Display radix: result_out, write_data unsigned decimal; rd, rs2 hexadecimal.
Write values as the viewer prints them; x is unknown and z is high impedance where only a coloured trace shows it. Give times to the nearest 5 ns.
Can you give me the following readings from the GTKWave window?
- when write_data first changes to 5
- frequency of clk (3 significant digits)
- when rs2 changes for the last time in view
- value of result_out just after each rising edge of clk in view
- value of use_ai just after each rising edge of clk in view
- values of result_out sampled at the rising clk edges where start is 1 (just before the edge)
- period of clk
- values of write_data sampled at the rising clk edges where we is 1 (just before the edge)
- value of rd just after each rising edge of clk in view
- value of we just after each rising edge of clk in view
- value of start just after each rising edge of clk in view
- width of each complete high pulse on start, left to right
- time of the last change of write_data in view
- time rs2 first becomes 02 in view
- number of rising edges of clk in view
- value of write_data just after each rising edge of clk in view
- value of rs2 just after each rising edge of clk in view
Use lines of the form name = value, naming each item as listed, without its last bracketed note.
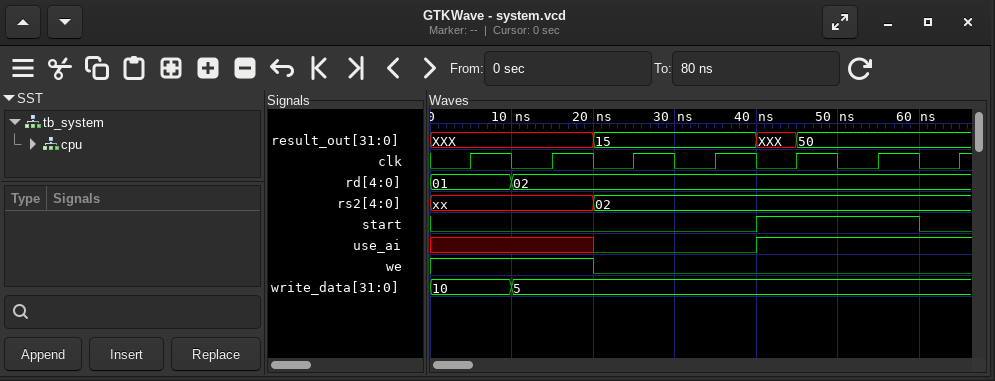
when write_data first changes to 5 = 10 ns
frequency of clk = 100 MHz
when rs2 changes for the last time in view = 20 ns
value of result_out just after each rising edge of clk in view = XXX, XXX, 15, 15, 50, 50, 50
value of use_ai just after each rising edge of clk in view = x x 0 0 1 1 1
values of result_out sampled at the rising clk edges where start is 1 = XXX, 50
period of clk = 10 ns
values of write_data sampled at the rising clk edges where we is 1 = 10, 5
value of rd just after each rising edge of clk in view = 01, 02, 02, 02, 02, 02, 02
value of we just after each rising edge of clk in view = 1 1 0 0 0 0 0
value of start just after each rising edge of clk in view = 0 0 0 0 1 1 0
width of each complete high pulse on start, left to right = 20 ns
time of the last change of write_data in view = 10 ns
time rs2 first becomes 02 in view = 20 ns
number of rising edges of clk in view = 7
value of write_data just after each rising edge of clk in view = 10, 5, 5, 5, 5, 5, 5
value of rs2 just after each rising edge of clk in view = xx, xx, 02, 02, 02, 02, 02
